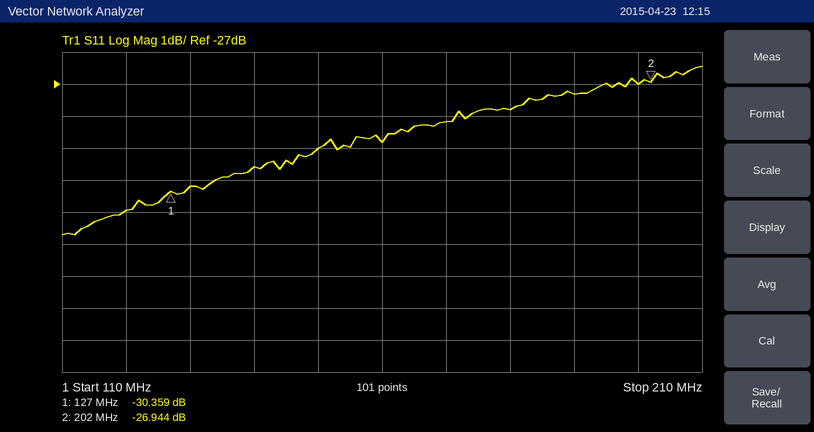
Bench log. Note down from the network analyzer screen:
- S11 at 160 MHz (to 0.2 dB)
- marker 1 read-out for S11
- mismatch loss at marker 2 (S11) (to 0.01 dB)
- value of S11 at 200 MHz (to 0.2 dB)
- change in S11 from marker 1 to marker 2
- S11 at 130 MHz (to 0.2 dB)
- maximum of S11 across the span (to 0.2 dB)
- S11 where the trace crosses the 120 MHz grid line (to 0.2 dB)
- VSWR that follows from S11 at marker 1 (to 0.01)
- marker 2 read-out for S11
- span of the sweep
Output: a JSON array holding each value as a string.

["-28.8 dB", "-30.359 dB", "0.01 dB", "-27.0 dB", "3.415 dB", "-30.2 dB", "-26.4 dB", "-31.0 dB", "1.06", "-26.944 dB", "100 MHz"]
